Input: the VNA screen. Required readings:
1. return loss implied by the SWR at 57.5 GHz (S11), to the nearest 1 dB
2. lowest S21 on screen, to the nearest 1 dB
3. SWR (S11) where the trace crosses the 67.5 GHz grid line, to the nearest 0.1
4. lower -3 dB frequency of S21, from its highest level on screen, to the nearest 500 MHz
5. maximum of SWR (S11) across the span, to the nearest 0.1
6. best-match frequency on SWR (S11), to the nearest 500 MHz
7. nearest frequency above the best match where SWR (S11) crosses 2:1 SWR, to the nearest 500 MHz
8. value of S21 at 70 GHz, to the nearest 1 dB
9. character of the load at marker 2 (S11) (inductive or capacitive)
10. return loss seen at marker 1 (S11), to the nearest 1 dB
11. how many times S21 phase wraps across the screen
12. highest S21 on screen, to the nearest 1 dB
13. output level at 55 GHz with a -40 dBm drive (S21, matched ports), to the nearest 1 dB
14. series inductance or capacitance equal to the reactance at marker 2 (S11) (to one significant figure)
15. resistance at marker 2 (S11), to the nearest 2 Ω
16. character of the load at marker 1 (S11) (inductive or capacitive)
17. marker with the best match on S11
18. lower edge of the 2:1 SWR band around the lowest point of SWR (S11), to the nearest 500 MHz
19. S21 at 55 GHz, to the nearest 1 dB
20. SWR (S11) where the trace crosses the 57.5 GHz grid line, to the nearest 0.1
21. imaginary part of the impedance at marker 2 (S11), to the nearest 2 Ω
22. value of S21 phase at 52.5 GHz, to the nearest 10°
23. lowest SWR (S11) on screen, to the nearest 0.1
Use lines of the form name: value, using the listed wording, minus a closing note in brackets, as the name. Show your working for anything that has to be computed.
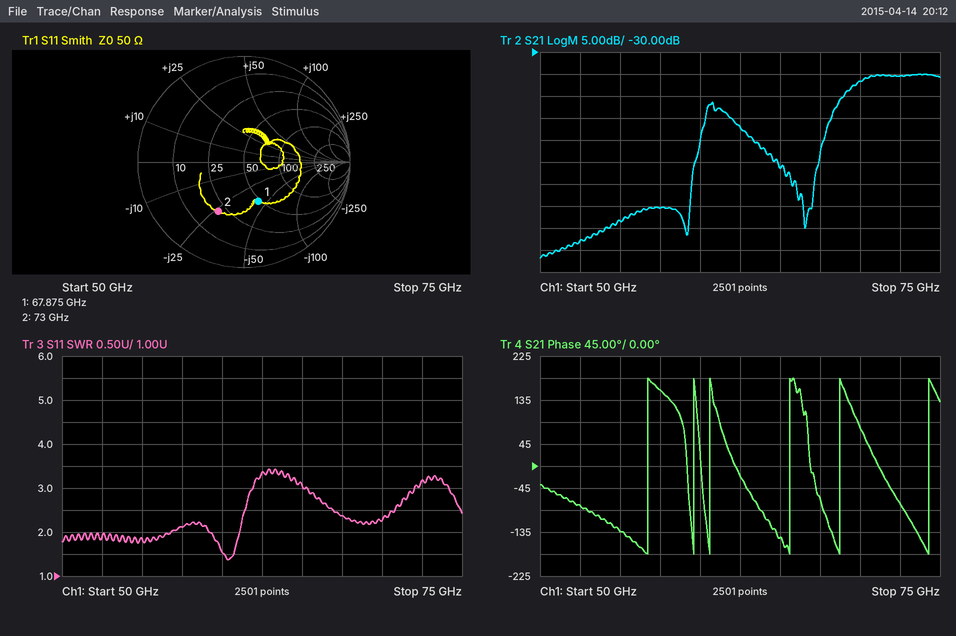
return loss implied by the SWR at 57.5 GHz (S11), to the nearest 1 dB: −20 log10((2.1 − 1)/(2.1 + 1)) ≈ 9 dB
lowest S21 on screen, to the nearest 1 dB: -77 dB
SWR (S11) where the trace crosses the 67.5 GHz grid line, to the nearest 0.1: 2.4
lower -3 dB frequency of S21, from its highest level on screen, to the nearest 500 MHz: 69.5 GHz
maximum of SWR (S11) across the span, to the nearest 0.1: 3.4
best-match frequency on SWR (S11), to the nearest 500 MHz: 60.5 GHz
nearest frequency above the best match where SWR (S11) crosses 2:1 SWR, to the nearest 500 MHz: 61.0 GHz
value of S21 at 70 GHz, to the nearest 1 dB: -37 dB
character of the load at marker 2 (S11): capacitive
return loss seen at marker 1 (S11), to the nearest 1 dB: 8 dB
how many times S21 phase wraps across the screen: 6
highest S21 on screen, to the nearest 1 dB: -35 dB
output level at 55 GHz with a -40 dBm drive (S21, matched ports), to the nearest 1 dB: -40 dBm + (-68 dB) = -108 dBm
series inductance or capacitance equal to the reactance at marker 2 (S11): C = 1/(2π × 73 GHz × 26 Ω) ≈ 83.9 fF, so 80 fF to one significant figure
resistance at marker 2 (S11), to the nearest 2 Ω: 20 Ω
character of the load at marker 1 (S11): capacitive
marker with the best match on S11: marker 1
lower edge of the 2:1 SWR band around the lowest point of SWR (S11), to the nearest 500 MHz: 59.0 GHz
S21 at 55 GHz, to the nearest 1 dB: -68 dB
SWR (S11) where the trace crosses the 57.5 GHz grid line, to the nearest 0.1: 2.1
imaginary part of the impedance at marker 2 (S11), to the nearest 2 Ω: -26 Ω
value of S21 phase at 52.5 GHz, to the nearest 10°: -80°
lowest SWR (S11) on screen, to the nearest 0.1: 1.4
